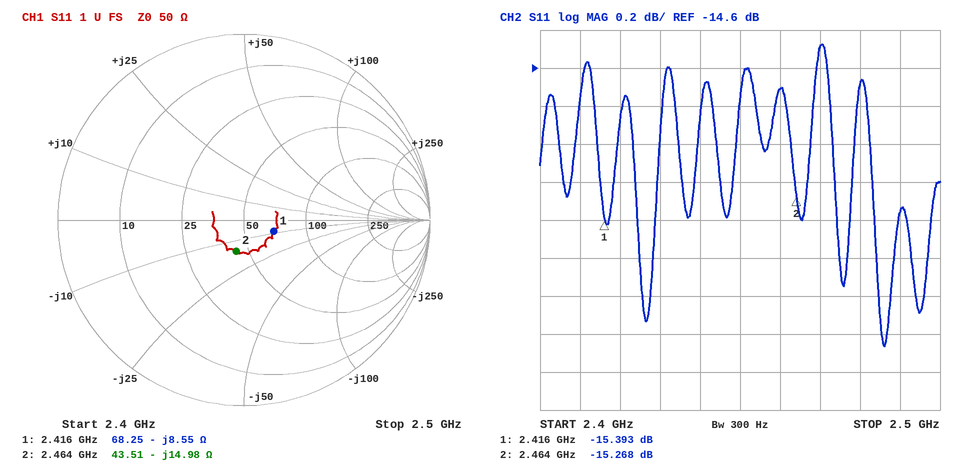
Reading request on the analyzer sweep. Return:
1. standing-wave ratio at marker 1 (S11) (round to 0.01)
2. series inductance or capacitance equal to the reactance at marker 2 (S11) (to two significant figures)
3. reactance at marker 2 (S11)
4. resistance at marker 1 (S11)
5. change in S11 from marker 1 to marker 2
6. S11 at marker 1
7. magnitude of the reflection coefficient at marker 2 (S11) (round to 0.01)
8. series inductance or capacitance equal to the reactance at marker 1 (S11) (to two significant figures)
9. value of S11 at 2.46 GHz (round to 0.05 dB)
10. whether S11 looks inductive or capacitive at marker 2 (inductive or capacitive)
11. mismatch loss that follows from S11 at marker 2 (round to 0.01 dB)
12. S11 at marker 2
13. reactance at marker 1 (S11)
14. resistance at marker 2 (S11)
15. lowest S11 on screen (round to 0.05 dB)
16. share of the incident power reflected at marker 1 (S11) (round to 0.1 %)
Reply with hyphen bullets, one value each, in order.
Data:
- 1.41
- 4.3 pF
- -14.98 Ω
- 68.25 Ω
- 0.125 dB
- -15.393 dB
- 0.17
- 7.7 pF
- -14.70 dB
- capacitive
- 0.13 dB
- -15.268 dB
- -8.55 Ω
- 43.51 Ω
- -16.05 dB
- 2.9 %
